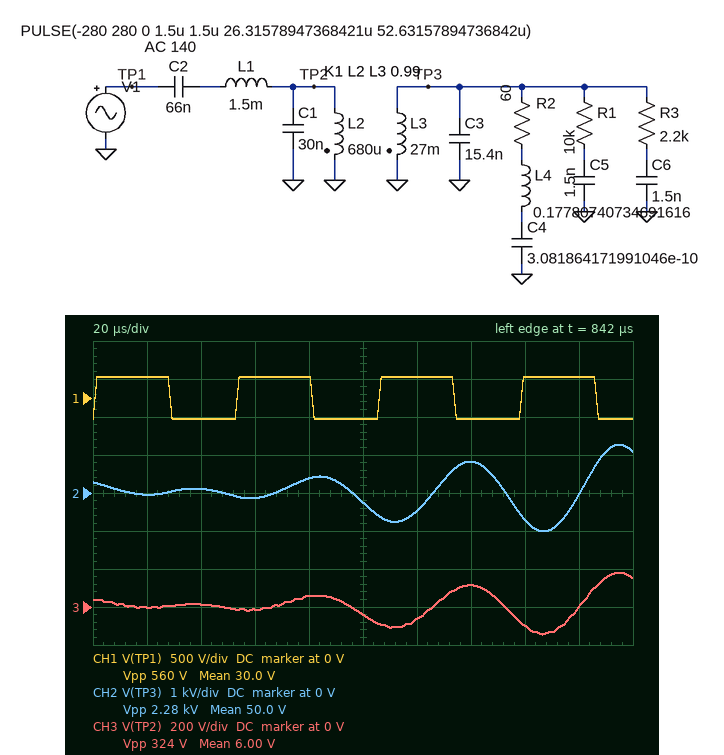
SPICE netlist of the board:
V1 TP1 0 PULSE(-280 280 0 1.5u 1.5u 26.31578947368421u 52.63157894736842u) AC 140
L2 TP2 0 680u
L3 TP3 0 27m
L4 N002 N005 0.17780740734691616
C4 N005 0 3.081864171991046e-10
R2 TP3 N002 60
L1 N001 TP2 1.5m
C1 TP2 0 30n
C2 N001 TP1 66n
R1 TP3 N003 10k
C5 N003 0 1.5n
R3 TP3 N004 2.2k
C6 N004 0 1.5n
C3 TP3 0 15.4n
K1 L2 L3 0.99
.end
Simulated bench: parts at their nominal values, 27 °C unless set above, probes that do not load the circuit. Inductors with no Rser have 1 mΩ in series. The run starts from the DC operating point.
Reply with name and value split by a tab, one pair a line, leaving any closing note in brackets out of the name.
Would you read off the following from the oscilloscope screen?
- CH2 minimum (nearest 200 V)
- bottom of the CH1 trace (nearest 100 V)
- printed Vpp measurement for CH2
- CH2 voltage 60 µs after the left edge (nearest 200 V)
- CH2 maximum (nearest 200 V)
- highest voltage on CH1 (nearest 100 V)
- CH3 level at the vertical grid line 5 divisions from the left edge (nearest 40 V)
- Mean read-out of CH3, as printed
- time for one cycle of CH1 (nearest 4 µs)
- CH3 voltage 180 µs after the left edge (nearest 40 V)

CH2 minimum	-1.0 kV
bottom of the CH1 trace	-300 V
printed Vpp measurement for CH2	2.28 kV
CH2 voltage 60 µs after the left edge	-200 V
CH2 maximum	1.2 kV
highest voltage on CH1	300 V
CH3 level at the vertical grid line 5 divisions from the left edge	-40 V
Mean read-out of CH3, as printed	6.00 V
time for one cycle of CH1	52 µs
CH3 voltage 180 µs after the left edge	0 V
